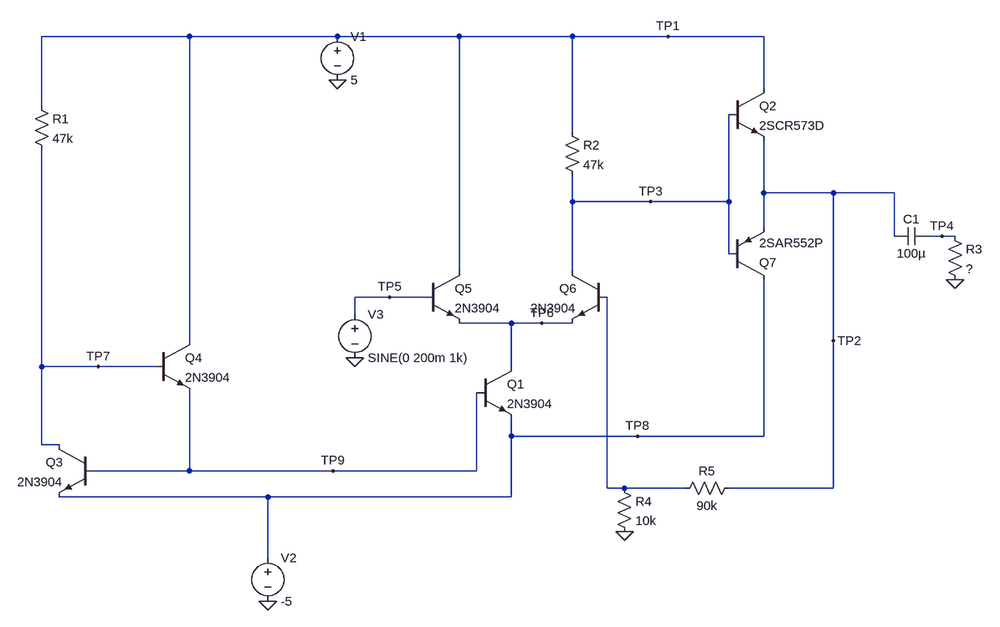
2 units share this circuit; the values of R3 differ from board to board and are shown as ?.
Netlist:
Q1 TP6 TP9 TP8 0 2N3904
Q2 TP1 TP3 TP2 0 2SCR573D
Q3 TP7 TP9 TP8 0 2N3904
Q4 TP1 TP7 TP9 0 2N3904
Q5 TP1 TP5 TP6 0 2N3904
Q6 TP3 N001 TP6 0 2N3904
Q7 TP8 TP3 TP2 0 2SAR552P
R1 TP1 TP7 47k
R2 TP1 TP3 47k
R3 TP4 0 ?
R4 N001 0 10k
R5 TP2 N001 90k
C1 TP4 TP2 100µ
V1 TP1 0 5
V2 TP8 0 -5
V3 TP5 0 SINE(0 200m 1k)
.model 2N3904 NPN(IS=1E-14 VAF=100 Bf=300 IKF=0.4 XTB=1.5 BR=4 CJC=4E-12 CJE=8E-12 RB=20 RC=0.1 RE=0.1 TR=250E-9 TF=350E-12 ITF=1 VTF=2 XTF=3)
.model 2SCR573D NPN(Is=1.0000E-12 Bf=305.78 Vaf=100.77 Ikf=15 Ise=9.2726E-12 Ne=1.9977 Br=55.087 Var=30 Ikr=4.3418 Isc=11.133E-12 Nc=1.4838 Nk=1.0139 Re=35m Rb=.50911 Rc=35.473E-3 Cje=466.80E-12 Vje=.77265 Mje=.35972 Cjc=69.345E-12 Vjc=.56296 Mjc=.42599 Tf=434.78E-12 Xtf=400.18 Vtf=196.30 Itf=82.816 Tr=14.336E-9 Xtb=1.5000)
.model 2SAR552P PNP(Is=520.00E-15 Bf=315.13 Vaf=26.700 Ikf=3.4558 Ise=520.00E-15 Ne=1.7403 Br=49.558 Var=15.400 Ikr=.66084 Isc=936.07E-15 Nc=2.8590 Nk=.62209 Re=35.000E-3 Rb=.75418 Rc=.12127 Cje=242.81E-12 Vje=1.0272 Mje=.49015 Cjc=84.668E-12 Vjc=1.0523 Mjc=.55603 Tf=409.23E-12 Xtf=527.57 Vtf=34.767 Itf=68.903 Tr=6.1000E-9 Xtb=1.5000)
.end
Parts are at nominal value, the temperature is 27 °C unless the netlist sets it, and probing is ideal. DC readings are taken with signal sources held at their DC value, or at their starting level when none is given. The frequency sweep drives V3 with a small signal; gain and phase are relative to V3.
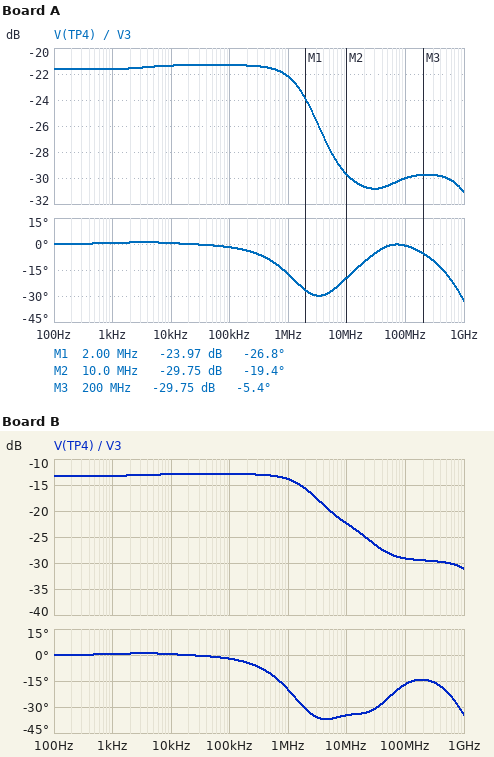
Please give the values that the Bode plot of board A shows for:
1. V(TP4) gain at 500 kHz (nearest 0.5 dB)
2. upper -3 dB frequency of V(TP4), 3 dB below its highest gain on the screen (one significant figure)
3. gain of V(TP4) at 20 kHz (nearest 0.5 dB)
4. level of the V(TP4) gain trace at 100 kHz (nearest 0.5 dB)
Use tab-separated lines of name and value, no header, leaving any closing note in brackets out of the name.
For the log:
V(TP4) gain at 500 kHz	-21.5 dB
upper -3 dB frequency of V(TP4), 3 dB below its highest gain on the screen	2 MHz
gain of V(TP4) at 20 kHz	-21.5 dB
level of the V(TP4) gain trace at 100 kHz	-21.5 dB
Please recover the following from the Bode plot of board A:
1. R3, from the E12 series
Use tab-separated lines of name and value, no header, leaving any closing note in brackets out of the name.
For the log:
R3, from the E12 series	56 Ω
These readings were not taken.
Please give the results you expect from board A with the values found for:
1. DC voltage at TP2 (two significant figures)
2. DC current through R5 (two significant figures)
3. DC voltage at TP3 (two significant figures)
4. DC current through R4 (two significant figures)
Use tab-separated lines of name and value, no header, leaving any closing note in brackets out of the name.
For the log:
DC voltage at TP2	45 mV
DC current through R5	480 nA
DC voltage at TP3	380 mV
DC current through R4	150 nA
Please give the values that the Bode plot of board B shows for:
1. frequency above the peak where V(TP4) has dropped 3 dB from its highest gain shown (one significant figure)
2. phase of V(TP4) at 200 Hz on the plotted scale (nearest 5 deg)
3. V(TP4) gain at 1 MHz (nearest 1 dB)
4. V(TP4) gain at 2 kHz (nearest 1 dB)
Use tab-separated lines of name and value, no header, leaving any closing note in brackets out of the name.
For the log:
frequency above the peak where V(TP4) has dropped 3 dB from its highest gain shown	2 MHz
phase of V(TP4) at 200 Hz on the plotted scale	0 deg
V(TP4) gain at 1 MHz	-14 dB
V(TP4) gain at 2 kHz	-13 dB
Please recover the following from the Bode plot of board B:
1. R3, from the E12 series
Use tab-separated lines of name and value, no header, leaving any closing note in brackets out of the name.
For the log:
R3, from the E12 series	150 Ω
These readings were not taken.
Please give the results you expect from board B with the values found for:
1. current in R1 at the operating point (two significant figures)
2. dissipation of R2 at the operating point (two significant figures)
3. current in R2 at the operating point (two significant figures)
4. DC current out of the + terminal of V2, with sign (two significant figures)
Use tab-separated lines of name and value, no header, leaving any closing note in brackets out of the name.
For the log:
current in R1 at the operating point	190 µA
dissipation of R2 at the operating point	450 µW
current in R2 at the operating point	98 µA
DC current out of the + terminal of V2, with sign	-390 µA
